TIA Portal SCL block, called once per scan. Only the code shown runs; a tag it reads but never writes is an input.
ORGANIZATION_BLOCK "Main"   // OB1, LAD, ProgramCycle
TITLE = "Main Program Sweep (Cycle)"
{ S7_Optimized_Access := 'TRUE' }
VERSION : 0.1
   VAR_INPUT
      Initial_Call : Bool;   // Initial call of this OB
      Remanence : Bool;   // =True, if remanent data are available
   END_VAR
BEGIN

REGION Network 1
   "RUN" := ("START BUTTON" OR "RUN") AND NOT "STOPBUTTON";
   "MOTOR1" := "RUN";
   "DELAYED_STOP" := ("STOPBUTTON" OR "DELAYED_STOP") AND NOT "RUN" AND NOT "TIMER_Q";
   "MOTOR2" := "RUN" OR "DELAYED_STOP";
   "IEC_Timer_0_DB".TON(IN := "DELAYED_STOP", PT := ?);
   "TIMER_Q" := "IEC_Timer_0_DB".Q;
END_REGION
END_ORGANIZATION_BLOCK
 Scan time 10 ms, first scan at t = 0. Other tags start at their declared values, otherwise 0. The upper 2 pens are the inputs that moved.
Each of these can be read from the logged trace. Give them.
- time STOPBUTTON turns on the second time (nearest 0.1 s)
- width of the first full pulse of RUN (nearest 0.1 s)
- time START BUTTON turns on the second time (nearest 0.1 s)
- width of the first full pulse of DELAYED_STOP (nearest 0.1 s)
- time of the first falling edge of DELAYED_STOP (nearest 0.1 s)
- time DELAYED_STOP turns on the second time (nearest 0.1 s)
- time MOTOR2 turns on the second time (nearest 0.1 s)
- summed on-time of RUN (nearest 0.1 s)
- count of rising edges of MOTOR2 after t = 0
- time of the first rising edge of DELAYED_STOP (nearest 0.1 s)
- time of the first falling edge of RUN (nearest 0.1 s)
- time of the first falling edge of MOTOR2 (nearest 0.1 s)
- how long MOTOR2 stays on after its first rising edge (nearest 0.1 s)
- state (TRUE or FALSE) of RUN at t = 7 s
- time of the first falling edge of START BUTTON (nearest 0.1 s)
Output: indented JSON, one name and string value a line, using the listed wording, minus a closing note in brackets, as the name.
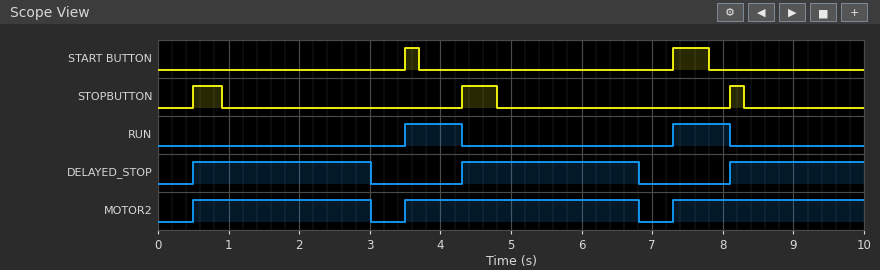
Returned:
{
  "time STOPBUTTON turns on the second time": "4.3 s",
  "width of the first full pulse of RUN": "0.8 s",
  "time START BUTTON turns on the second time": "7.3 s",
  "width of the first full pulse of DELAYED_STOP": "2.5 s",
  "time of the first falling edge of DELAYED_STOP": "3.0 s",
  "time DELAYED_STOP turns on the second time": "4.3 s",
  "time MOTOR2 turns on the second time": "3.5 s",
  "summed on-time of RUN": "1.6 s",
  "count of rising edges of MOTOR2 after t = 0": "3",
  "time of the first rising edge of DELAYED_STOP": "0.5 s",
  "time of the first falling edge of RUN": "4.3 s",
  "time of the first falling edge of MOTOR2": "3.0 s",
  "how long MOTOR2 stays on after its first rising edge": "2.5 s",
  "state (TRUE or FALSE) of RUN at t = 7 s": "FALSE",
  "time of the first falling edge of START BUTTON": "3.7 s"
}
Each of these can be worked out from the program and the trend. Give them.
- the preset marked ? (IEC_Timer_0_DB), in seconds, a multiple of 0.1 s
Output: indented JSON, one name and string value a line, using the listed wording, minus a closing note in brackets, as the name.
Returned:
{
  "the preset marked ? (IEC_Timer_0_DB), in seconds, a multiple of 0.1 s": "2.5 s"
}
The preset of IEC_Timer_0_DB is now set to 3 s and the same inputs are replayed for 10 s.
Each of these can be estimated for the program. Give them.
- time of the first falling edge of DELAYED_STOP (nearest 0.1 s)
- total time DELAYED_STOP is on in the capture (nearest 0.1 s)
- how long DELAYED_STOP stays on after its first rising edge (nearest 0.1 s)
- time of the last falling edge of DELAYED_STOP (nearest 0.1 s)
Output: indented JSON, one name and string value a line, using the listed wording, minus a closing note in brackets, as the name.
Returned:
{
  "time of the first falling edge of DELAYED_STOP": "3.5 s",
  "total time DELAYED_STOP is on in the capture": "7.9 s",
  "how long DELAYED_STOP stays on after its first rising edge": "3.0 s",
  "time of the last falling edge of DELAYED_STOP": "7.3 s"
}
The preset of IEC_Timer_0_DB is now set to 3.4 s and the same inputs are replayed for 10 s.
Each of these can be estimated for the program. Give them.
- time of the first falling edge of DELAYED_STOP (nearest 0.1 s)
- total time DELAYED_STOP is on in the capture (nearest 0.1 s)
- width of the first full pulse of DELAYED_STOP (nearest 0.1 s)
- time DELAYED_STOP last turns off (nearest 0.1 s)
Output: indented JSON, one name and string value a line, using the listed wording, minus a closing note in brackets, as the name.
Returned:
{
  "time of the first falling edge of DELAYED_STOP": "3.5 s",
  "total time DELAYED_STOP is on in the capture": "7.9 s",
  "width of the first full pulse of DELAYED_STOP": "3.0 s",
  "time DELAYED_STOP last turns off": "7.3 s"
}
